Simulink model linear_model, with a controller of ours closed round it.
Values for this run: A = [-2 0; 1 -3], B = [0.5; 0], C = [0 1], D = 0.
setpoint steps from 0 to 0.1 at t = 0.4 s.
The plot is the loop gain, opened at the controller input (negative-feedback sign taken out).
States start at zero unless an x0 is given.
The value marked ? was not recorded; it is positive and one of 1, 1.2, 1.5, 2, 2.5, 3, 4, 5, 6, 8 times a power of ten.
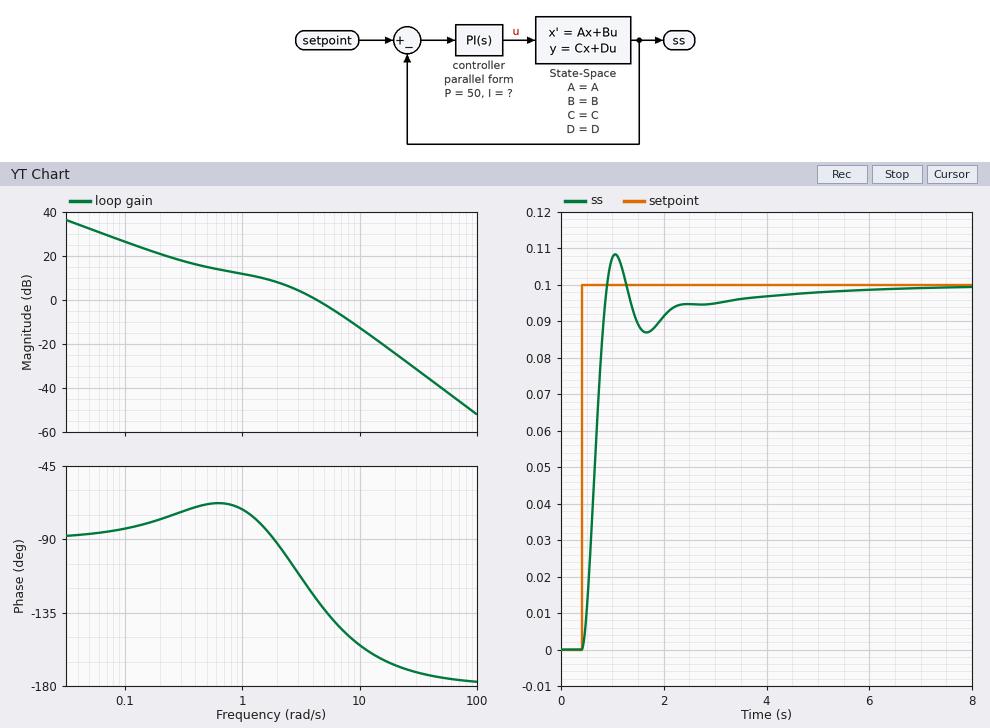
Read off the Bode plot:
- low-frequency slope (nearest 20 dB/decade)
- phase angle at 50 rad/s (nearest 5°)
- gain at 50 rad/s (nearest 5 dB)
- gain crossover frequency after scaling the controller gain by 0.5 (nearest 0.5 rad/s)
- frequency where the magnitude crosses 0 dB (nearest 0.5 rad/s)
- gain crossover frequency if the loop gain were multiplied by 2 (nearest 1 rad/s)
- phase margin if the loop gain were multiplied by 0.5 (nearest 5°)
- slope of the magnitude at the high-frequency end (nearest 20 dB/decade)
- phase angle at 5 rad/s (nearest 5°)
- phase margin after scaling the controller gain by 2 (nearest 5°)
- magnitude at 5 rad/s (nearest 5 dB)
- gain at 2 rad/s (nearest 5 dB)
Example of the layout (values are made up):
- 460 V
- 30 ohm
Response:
- -20 dB/decade
- -175°
- -40 dB
- 2.5 rad/s
- 4.5 rad/s
- 7 rad/s
- 75°
- -40 dB/decade
- -135°
- 35°
- 0 dB
- 10 dB
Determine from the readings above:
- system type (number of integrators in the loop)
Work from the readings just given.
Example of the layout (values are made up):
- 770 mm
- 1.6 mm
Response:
- 1
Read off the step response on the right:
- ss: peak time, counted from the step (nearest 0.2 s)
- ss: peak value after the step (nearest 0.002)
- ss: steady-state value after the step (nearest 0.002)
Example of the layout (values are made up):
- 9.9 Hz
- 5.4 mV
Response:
- 0.6 s
- 0.108
- 0.100
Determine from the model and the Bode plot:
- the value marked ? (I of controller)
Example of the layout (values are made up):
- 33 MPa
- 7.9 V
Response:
- 25
